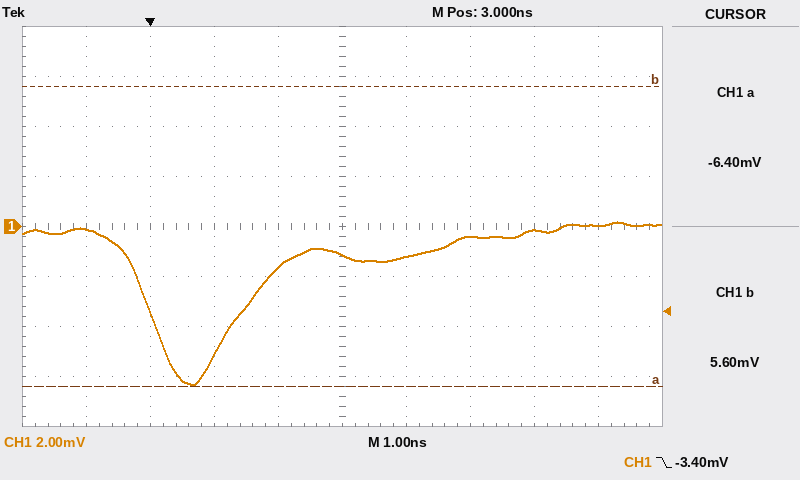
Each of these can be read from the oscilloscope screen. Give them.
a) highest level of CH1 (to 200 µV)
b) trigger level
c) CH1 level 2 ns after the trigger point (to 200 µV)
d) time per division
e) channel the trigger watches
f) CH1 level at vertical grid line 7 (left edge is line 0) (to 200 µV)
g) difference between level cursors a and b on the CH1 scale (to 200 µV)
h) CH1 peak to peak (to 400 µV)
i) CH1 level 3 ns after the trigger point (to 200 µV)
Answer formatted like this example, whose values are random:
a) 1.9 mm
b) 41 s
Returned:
a) 200 µV
b) -3.40 mV
c) -1.6 mV
d) 1 ns
e) CH1
f) -400 µV
g) 12.0 mV
h) 6.4 mV
i) -1.2 mV
